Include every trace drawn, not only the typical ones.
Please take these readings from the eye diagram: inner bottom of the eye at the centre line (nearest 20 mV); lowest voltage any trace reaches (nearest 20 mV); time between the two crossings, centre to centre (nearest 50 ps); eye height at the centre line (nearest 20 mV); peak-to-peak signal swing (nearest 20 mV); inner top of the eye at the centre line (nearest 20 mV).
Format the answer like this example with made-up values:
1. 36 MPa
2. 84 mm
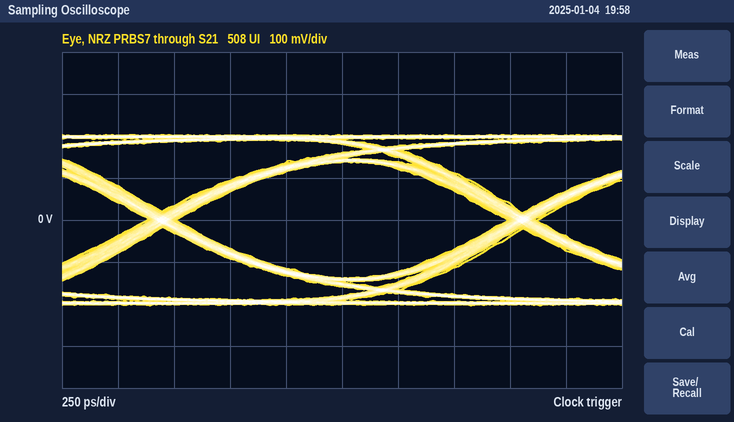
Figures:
1. -140 mV
2. -200 mV
3. 1.60 ns
4. 280 mV
5. 400 mV
6. 140 mV
